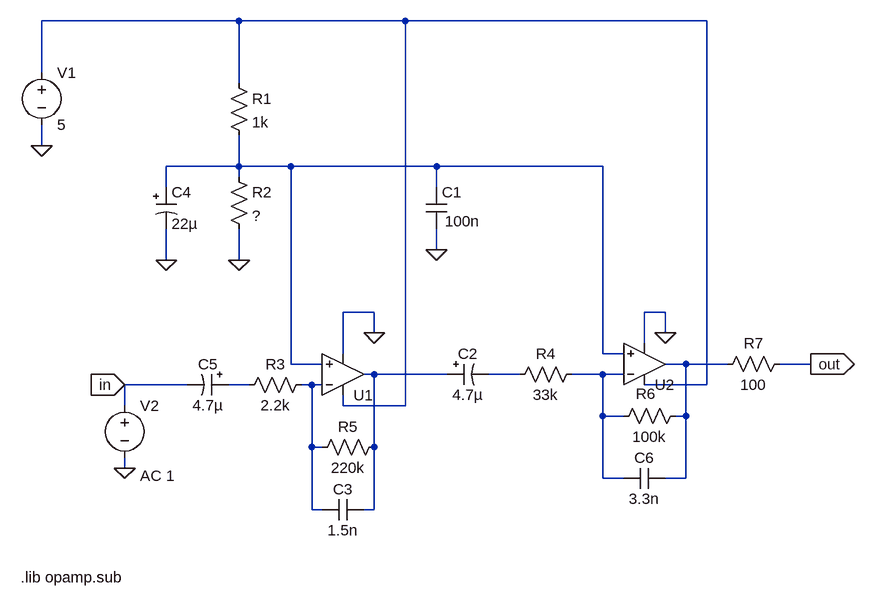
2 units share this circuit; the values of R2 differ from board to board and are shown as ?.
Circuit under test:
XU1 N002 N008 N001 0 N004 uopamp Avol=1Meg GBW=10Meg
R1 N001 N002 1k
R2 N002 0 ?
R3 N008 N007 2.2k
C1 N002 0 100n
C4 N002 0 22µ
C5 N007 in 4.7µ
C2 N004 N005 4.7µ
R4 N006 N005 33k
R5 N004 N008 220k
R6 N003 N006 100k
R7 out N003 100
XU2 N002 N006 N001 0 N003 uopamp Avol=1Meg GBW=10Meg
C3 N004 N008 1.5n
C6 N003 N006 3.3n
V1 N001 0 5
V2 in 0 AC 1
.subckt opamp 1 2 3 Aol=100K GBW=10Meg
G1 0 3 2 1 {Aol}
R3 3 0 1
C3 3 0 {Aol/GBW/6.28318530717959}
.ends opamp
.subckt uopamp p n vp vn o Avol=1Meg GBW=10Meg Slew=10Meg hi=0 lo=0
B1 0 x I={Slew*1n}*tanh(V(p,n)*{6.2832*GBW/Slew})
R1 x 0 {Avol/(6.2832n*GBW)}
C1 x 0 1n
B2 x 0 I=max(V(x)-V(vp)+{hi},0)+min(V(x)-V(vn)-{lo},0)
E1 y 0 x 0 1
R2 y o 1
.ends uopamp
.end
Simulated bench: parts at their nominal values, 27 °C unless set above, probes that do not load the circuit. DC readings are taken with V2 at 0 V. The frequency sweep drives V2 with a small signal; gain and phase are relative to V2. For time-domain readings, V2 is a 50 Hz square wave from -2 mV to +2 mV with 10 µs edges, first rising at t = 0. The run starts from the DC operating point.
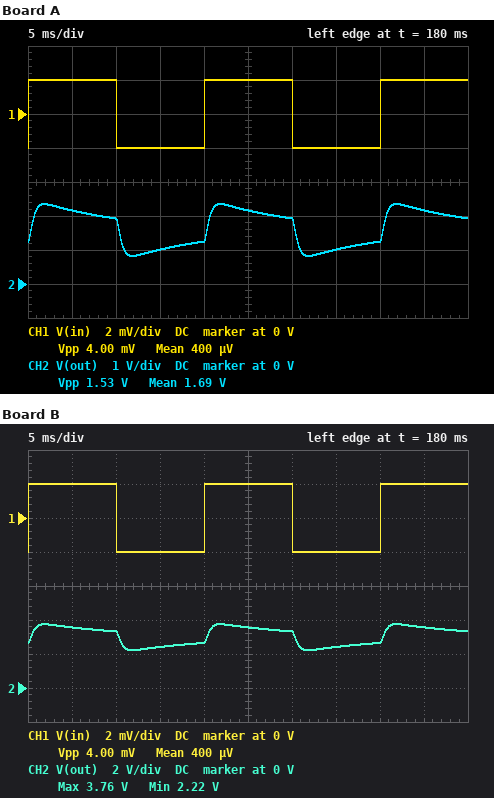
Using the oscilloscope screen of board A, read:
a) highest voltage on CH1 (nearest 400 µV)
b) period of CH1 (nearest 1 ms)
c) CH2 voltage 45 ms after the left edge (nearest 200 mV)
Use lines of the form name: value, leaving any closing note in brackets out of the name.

highest voltage on CH1: 2.0 mV
period of CH1: 20 ms
CH2 voltage 45 ms after the left edge: 2.2 V
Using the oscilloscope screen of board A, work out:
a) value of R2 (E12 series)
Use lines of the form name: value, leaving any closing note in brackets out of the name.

value of R2: 470 Ω
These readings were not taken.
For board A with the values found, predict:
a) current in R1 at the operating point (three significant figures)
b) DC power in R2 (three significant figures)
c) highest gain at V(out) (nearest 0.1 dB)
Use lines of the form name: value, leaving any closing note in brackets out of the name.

current in R1 at the operating point: 3.40 mA
DC power in R2: 5.44 mW
highest gain at V(out): 49.2 dB
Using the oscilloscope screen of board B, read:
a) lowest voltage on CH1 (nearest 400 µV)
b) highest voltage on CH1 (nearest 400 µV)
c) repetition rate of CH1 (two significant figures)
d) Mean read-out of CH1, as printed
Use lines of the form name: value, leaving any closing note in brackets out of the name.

lowest voltage on CH1: -2.0 mV
highest voltage on CH1: 2.0 mV
repetition rate of CH1: 50 Hz
Mean read-out of CH1, as printed: 400 µV
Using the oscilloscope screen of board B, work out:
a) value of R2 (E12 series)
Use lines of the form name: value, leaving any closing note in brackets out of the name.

value of R2: 1.5 kΩ
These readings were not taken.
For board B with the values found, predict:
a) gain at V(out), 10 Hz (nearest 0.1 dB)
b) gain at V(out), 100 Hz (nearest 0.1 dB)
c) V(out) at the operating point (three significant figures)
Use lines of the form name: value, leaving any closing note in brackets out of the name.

gain at V(out), 10 Hz: 44.3 dB
gain at V(out), 100 Hz: 49.2 dB
V(out) at the operating point: 3.00 V
